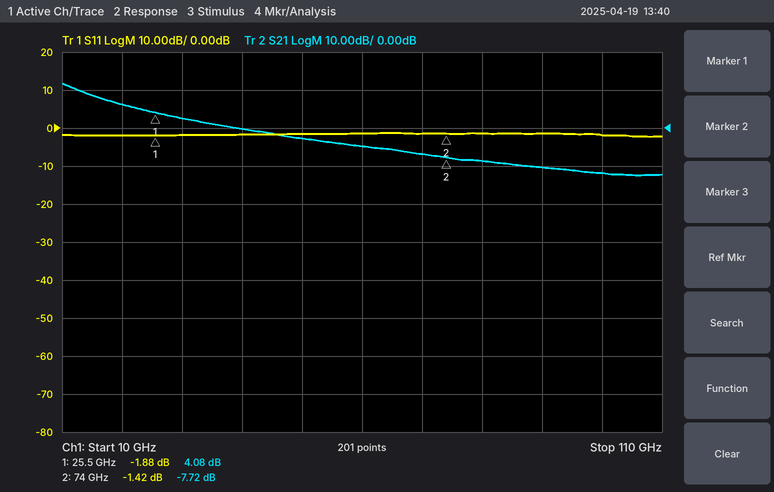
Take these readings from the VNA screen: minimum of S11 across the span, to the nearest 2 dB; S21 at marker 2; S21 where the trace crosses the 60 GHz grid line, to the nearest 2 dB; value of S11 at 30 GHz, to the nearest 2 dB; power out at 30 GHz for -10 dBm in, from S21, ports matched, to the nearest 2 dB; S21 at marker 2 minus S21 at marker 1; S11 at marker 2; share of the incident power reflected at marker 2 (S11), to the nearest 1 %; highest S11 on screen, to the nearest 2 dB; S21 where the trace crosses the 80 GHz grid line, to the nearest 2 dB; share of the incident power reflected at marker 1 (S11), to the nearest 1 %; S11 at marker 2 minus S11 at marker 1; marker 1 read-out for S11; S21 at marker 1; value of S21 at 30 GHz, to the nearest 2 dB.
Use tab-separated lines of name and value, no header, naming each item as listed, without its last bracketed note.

minimum of S11 across the span, to the nearest 2 dB	-2 dB
S21 at marker 2	-7.72 dB
S21 where the trace crosses the 60 GHz grid line, to the nearest 2 dB	-4 dB
value of S11 at 30 GHz, to the nearest 2 dB	-2 dB
power out at 30 GHz for -10 dBm in, from S21, ports matched, to the nearest 2 dB	-8 dBm
S21 at marker 2 minus S21 at marker 1	-11.80 dB
S11 at marker 2	-1.42 dB
share of the incident power reflected at marker 2 (S11), to the nearest 1 %	72 %
highest S11 on screen, to the nearest 2 dB	-2 dB
S21 where the trace crosses the 80 GHz grid line, to the nearest 2 dB	-8 dB
share of the incident power reflected at marker 1 (S11), to the nearest 1 %	65 %
S11 at marker 2 minus S11 at marker 1	0.46 dB
marker 1 read-out for S11	-1.88 dB
S21 at marker 1	4.08 dB
value of S21 at 30 GHz, to the nearest 2 dB	2 dB
